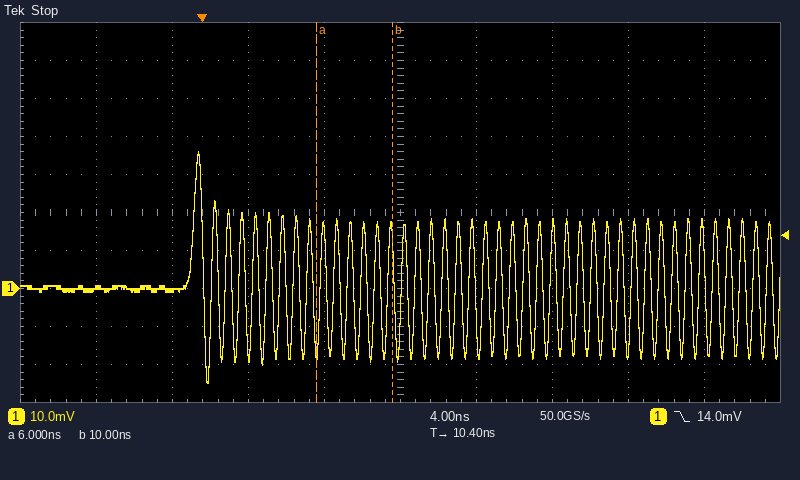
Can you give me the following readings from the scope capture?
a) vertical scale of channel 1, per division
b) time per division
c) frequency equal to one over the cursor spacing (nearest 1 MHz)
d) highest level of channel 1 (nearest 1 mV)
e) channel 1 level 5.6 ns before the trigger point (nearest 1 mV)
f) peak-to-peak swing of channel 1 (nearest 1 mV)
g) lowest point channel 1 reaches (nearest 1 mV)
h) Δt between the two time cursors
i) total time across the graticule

10 mV
4 ns
250 MHz
36 mV
0 mV
61 mV
-25 mV
4.0 ns
40 ns
